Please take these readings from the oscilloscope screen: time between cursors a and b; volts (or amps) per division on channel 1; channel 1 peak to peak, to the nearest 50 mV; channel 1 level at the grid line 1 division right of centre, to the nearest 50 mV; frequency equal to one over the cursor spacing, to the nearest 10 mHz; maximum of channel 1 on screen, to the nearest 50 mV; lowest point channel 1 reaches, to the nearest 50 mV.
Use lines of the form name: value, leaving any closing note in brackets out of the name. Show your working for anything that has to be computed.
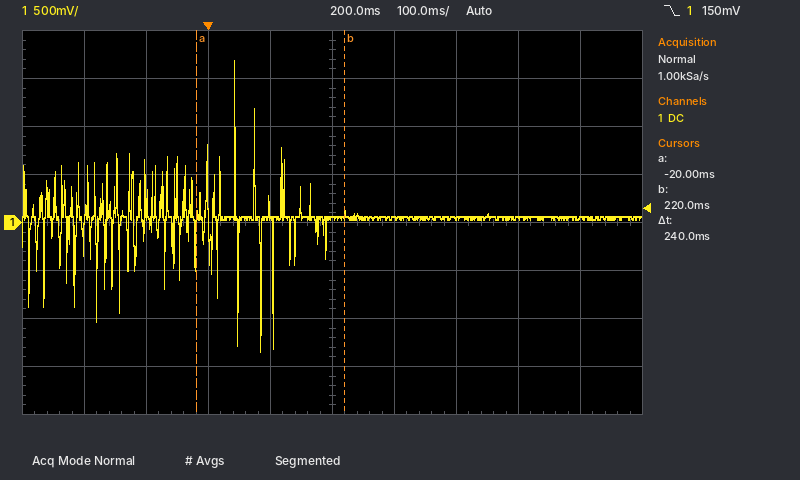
time between cursors a and b: 240 ms
volts (or amps) per division on channel 1: 500 mV
channel 1 peak to peak, to the nearest 50 mV: 1.70 V − (-1.35 V) = 3.05 V
channel 1 level at the grid line 1 division right of centre, to the nearest 50 mV: 50 mV
frequency equal to one over the cursor spacing, to the nearest 10 mHz: 1 / 240 ms ≈ 4.17 Hz
maximum of channel 1 on screen, to the nearest 50 mV: 1.70 V
lowest point channel 1 reaches, to the nearest 50 mV: -1.35 V
